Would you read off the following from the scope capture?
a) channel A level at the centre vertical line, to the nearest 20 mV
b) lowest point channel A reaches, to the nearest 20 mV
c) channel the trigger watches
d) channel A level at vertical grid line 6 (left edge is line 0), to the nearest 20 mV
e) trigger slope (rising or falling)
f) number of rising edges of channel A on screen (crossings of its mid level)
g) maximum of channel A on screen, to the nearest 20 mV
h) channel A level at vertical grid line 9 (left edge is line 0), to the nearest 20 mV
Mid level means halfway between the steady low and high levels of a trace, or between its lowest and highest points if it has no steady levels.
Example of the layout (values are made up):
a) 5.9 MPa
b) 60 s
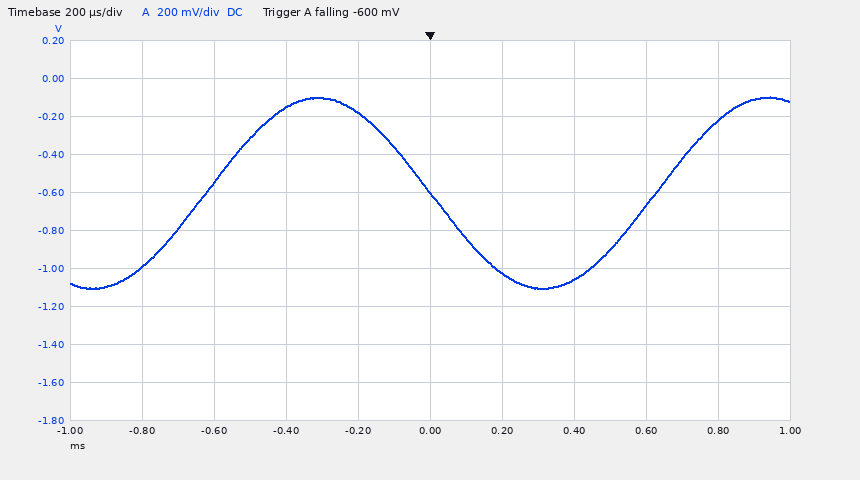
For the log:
a) -600 mV
b) -1.10 V
c) channel A
d) -1.02 V
e) falling
f) 2
g) -100 mV
h) -220 mV
